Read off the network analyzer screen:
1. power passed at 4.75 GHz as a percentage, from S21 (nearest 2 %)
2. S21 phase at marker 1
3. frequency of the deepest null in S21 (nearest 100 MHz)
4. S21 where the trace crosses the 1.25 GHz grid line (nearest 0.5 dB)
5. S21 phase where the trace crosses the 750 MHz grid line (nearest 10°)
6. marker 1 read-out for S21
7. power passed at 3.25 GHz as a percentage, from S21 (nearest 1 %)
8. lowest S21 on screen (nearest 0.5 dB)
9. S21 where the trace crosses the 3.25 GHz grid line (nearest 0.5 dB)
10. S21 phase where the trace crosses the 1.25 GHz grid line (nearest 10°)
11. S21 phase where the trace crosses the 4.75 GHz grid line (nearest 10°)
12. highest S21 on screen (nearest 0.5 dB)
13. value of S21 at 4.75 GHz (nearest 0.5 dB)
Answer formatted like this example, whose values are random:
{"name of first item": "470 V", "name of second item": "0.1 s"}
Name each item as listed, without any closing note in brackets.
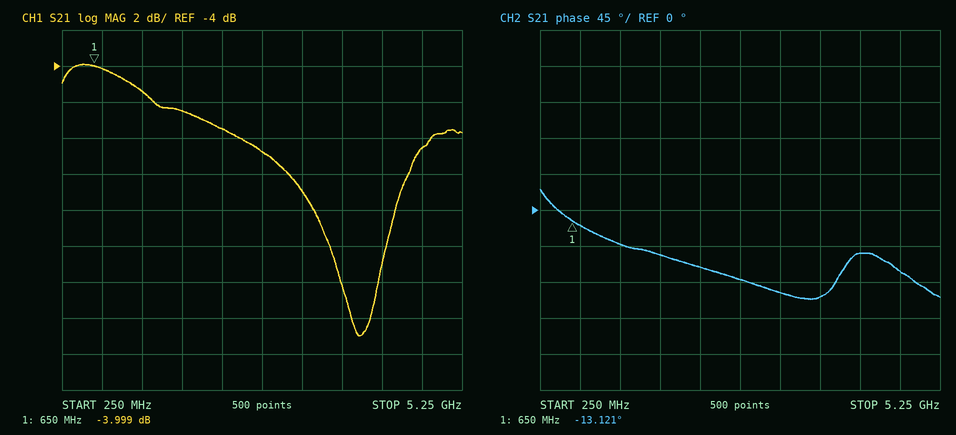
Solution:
{"power passed at 4.75 GHz as a percentage, from S21": "14 %", "S21 phase at marker 1": "-13.121°", "frequency of the deepest null in S21": "4.0 GHz", "S21 where the trace crosses the 1.25 GHz grid line": "-5.5 dB", "S21 phase where the trace crosses the 750 MHz grid line": "-20°", "marker 1 read-out for S21": "-3.999 dB", "power passed at 3.25 GHz as a percentage, from S21": "8 %", "lowest S21 on screen": "-19.0 dB", "S21 where the trace crosses the 3.25 GHz grid line": "-11.0 dB", "S21 phase where the trace crosses the 1.25 GHz grid line": "-40°", "S21 phase where the trace crosses the 4.75 GHz grid line": "-80°", "highest S21 on screen": "-4.0 dB", "value of S21 at 4.75 GHz": "-8.5 dB"}
